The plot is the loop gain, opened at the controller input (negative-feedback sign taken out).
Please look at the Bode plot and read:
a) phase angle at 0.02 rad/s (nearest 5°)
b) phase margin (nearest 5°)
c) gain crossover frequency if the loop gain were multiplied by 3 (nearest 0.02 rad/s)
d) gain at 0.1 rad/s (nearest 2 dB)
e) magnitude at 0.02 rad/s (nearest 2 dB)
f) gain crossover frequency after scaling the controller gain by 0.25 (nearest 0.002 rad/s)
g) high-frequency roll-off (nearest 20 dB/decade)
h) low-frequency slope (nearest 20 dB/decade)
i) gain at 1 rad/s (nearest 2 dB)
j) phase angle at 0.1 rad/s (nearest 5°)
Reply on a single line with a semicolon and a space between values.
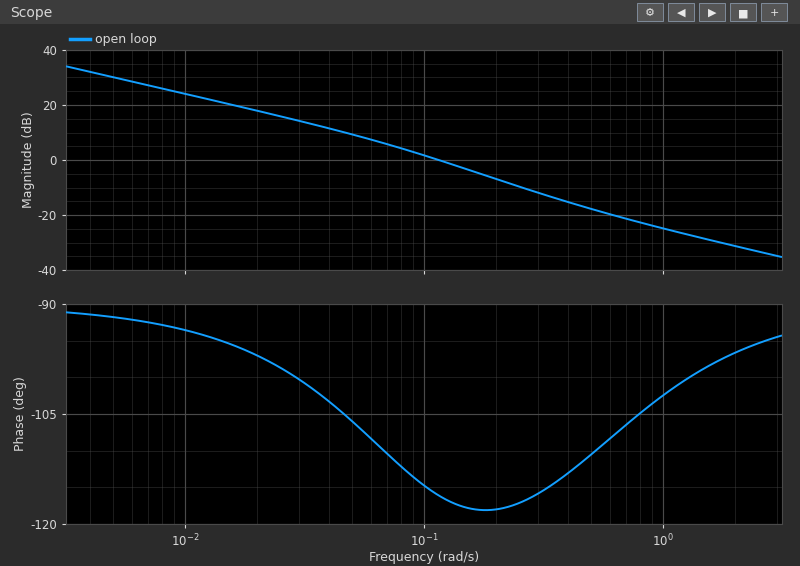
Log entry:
-95°; 65°; 0.24 rad/s; 2 dB; 18 dB; 0.038 rad/s; -20 dB/decade; -20 dB/decade; -24 dB; -115°
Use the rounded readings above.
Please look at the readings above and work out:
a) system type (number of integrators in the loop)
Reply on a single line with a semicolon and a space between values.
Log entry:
1
